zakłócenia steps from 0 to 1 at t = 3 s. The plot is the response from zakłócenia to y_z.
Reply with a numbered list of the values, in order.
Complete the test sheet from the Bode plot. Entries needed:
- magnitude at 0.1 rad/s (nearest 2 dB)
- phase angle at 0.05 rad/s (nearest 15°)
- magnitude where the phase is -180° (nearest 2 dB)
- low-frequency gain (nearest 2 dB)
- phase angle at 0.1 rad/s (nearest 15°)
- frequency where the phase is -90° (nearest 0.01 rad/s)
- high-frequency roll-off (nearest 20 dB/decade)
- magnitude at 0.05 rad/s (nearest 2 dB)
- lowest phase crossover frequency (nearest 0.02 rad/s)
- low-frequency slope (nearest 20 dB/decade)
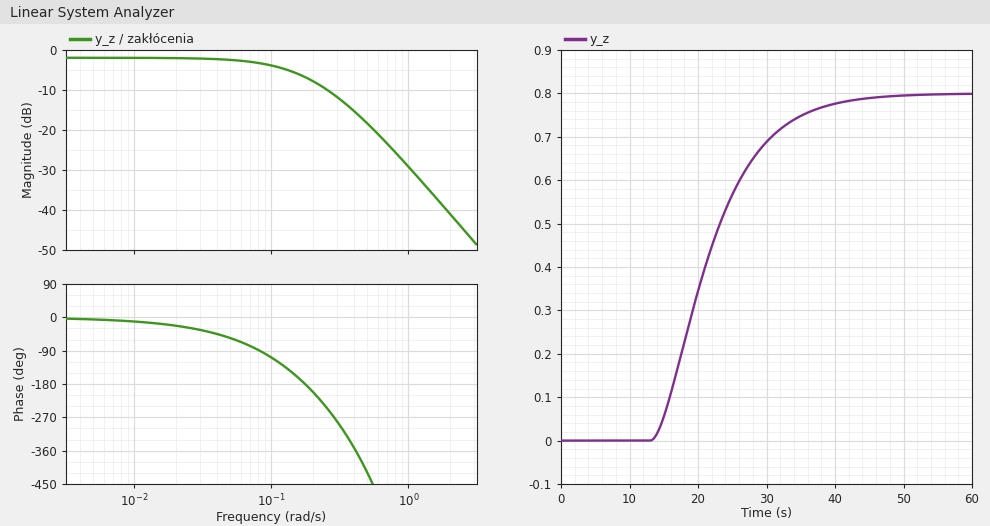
1. -4 dB
2. -60°
3. -6 dB
4. -2 dB
5. -105°
6. 0.08 rad/s
7. -40 dB/decade
8. -2 dB
9. 0.18 rad/s
10. 0 dB/decade
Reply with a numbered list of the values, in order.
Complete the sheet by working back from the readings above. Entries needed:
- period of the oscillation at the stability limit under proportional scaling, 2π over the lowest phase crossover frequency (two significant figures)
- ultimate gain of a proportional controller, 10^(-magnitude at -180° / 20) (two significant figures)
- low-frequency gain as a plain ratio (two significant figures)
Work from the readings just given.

1. 35 s
2. 2.0
3. 0.79
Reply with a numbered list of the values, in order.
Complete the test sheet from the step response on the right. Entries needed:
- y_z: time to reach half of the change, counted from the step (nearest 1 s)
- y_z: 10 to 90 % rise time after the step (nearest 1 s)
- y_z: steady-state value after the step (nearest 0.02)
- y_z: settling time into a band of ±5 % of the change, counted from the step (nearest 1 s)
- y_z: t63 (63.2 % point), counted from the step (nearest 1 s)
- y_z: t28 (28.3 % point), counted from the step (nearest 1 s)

1. 18 s
2. 17 s
3. 0.80
4. 34 s
5. 20 s
6. 15 s
